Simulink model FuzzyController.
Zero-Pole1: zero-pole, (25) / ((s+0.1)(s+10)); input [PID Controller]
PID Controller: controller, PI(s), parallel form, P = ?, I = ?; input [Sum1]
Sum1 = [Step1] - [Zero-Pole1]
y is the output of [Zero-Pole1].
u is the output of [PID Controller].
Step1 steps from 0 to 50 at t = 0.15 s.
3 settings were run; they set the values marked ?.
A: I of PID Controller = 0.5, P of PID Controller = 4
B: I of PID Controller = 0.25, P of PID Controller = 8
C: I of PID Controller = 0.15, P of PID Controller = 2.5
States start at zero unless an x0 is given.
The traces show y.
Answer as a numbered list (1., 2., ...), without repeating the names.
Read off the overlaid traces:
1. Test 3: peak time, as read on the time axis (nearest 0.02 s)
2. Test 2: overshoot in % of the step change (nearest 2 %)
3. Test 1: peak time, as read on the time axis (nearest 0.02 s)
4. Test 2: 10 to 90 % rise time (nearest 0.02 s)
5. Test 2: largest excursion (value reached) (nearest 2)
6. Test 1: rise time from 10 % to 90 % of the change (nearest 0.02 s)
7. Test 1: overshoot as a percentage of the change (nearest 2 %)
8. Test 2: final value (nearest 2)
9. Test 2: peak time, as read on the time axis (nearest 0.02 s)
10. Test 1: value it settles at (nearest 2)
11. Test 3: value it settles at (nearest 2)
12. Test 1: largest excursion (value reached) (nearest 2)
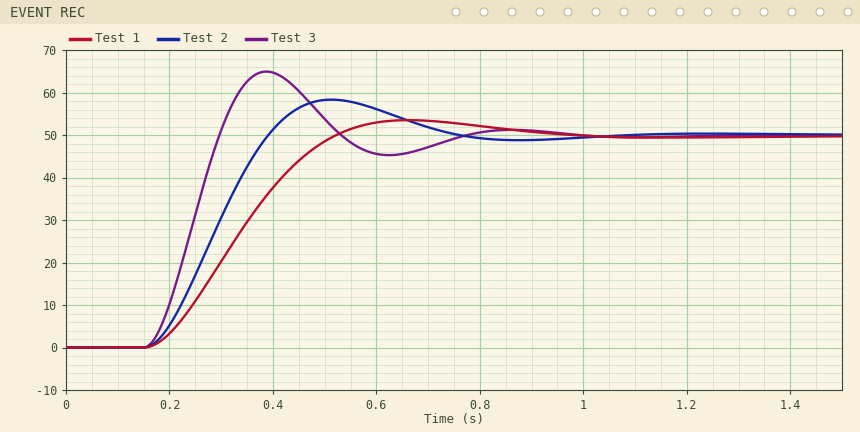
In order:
1. 0.38 s
2. 16 %
3. 0.66 s
4. 0.16 s
5. 58
6. 0.24 s
7. 8 %
8. 50
9. 0.52 s
10. 50
11. 50
12. 54
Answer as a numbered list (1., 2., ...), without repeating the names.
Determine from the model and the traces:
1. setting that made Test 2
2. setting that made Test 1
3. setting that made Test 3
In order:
1. A
2. C
3. B
